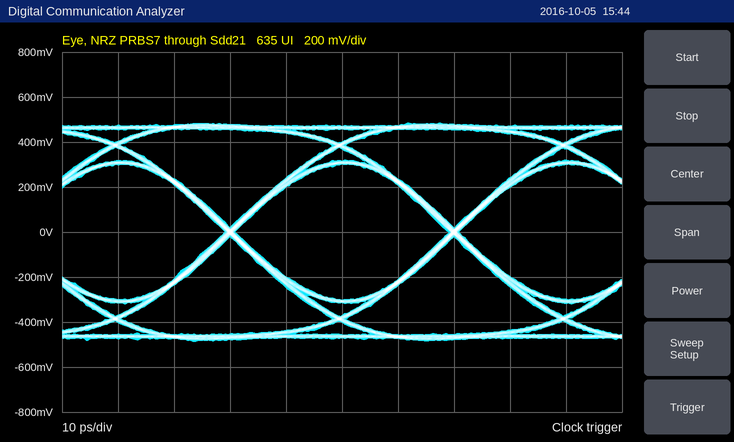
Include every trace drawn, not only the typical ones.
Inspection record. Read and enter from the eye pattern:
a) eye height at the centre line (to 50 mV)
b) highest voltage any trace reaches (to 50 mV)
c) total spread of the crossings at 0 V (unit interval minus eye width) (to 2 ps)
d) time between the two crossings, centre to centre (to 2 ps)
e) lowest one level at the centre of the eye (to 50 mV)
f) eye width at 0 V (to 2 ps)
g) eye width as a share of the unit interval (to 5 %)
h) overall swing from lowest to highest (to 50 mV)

600 mV
500 mV
2 ps
40 ps
300 mV
38 ps
95 %
950 mV
